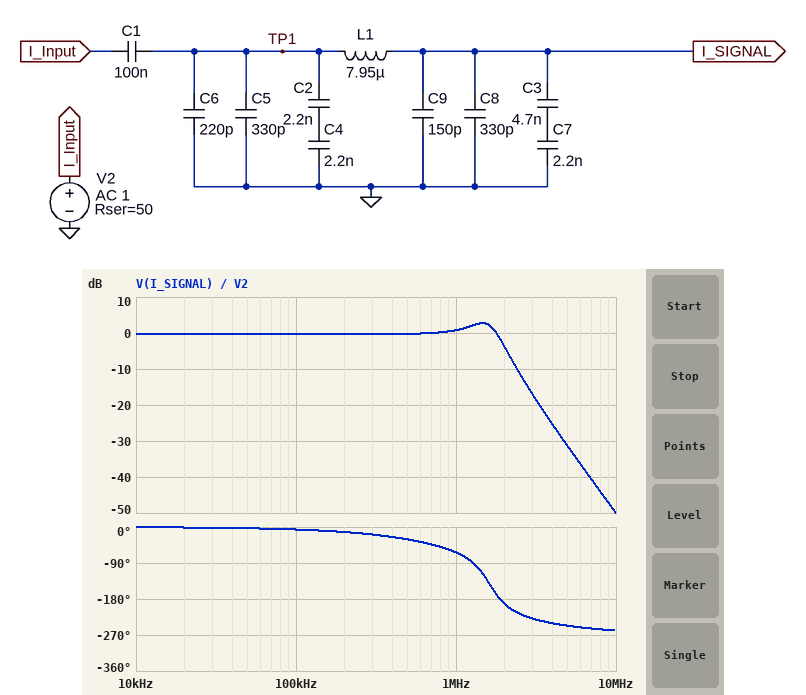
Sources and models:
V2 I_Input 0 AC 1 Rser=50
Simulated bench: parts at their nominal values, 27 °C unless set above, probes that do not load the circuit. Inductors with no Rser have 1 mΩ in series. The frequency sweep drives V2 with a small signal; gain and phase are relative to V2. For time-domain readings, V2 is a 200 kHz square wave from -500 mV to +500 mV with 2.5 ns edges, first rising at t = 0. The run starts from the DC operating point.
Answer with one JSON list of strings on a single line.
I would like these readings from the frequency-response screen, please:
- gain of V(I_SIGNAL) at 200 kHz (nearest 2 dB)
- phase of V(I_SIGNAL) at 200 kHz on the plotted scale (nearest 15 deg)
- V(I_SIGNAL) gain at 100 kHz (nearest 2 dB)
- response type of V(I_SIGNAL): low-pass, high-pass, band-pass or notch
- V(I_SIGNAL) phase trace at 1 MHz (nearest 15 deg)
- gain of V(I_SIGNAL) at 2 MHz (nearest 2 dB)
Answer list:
["0 dB", "-15 deg", "0 dB", "low-pass", "-60 deg", "-4 dB"]
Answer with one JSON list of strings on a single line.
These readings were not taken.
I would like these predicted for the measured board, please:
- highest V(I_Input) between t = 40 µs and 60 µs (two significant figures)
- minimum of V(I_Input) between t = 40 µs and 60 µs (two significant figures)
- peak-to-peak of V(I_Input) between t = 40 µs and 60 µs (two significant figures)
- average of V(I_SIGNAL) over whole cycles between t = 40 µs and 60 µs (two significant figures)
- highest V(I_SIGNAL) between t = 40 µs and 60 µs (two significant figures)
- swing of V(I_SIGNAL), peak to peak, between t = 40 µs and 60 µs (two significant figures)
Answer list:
["620 mV", "-620 mV", "1.2 V", "480 mV", "1.2 V", "1.4 V"]
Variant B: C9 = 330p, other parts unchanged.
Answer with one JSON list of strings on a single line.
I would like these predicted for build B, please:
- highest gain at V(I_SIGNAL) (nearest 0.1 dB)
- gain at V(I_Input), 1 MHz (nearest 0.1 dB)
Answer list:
["2.2 dB", "-8.4 dB"]
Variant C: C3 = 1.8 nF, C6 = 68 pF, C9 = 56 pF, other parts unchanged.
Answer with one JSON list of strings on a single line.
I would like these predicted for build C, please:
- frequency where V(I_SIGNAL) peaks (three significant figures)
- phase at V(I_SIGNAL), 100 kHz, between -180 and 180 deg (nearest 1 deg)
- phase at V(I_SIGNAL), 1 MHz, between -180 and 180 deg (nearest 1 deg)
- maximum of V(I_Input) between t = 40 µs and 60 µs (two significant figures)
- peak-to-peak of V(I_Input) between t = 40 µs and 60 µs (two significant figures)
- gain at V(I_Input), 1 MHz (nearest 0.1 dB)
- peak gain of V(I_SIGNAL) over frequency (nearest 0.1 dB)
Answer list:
["1.75 MHz", "-5 deg", "-50 deg", "630 mV", "1.3 V", "-3.8 dB", "4.7 dB"]
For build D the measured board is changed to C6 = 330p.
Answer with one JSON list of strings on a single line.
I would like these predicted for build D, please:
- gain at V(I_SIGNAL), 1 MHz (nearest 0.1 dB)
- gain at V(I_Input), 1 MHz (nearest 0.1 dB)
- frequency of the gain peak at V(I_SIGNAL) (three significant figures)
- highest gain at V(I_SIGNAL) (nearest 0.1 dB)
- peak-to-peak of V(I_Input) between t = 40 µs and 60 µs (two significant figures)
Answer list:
["0.7 dB", "-7.2 dB", "1.49 MHz", "2.9 dB", "1.2 V"]
